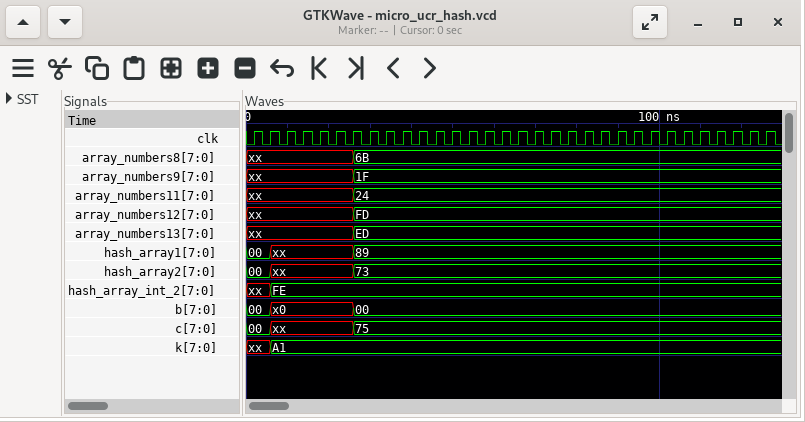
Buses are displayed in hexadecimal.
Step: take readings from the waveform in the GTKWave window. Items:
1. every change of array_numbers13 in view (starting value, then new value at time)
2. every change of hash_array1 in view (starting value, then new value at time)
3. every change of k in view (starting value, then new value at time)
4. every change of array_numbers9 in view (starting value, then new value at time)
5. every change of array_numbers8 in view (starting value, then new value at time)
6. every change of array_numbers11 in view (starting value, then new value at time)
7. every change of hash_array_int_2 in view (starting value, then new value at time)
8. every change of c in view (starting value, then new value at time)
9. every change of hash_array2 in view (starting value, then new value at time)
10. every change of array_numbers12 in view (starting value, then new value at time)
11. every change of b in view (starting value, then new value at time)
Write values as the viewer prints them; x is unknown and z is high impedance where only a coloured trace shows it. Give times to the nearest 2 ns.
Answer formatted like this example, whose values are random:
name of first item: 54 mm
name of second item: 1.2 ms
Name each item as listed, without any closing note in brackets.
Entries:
every change of array_numbers13 in view: xx, ED at 26 ns
every change of hash_array1 in view: 00, xx at 6 ns, 89 at 26 ns
every change of k in view: xx, A1 at 6 ns
every change of array_numbers9 in view: xx, 1F at 26 ns
every change of array_numbers8 in view: xx, 6B at 26 ns
every change of array_numbers11 in view: xx, 24 at 26 ns
every change of hash_array_int_2 in view: xx, FE at 6 ns
every change of c in view: 00, xx at 6 ns, 75 at 26 ns
every change of hash_array2 in view: 00, xx at 6 ns, 73 at 26 ns
every change of array_numbers12 in view: xx, FD at 26 ns
every change of b in view: 00, x0 at 6 ns, 00 at 26 ns
